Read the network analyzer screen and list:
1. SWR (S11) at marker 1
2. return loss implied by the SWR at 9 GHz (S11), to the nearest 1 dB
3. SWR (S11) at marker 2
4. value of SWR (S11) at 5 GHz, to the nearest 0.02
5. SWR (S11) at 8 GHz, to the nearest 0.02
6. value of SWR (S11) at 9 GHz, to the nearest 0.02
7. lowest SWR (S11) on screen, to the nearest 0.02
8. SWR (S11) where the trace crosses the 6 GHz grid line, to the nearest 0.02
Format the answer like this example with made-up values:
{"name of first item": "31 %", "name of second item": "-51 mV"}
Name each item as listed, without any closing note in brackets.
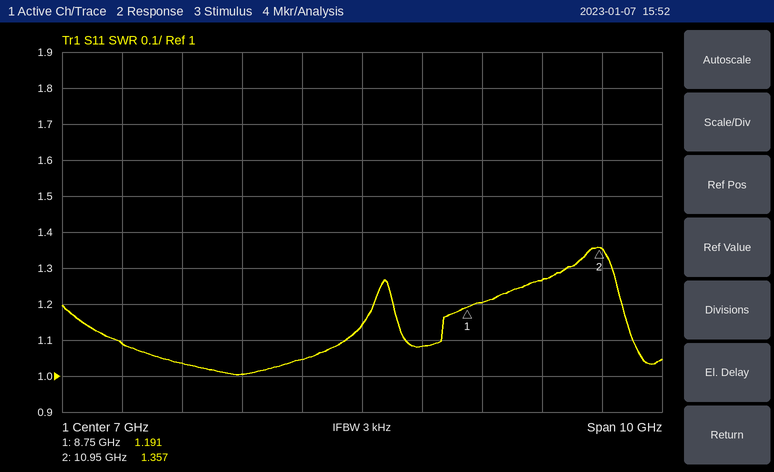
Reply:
{"SWR (S11) at marker 1": "1.191", "return loss implied by the SWR at 9 GHz (S11), to the nearest 1 dB": "21 dB", "SWR (S11) at marker 2": "1.357", "value of SWR (S11) at 5 GHz, to the nearest 0.02": "1.00", "SWR (S11) at 8 GHz, to the nearest 0.02": "1.08", "value of SWR (S11) at 9 GHz, to the nearest 0.02": "1.20", "lowest SWR (S11) on screen, to the nearest 0.02": "1.00", "SWR (S11) where the trace crosses the 6 GHz grid line, to the nearest 0.02": "1.04"}
